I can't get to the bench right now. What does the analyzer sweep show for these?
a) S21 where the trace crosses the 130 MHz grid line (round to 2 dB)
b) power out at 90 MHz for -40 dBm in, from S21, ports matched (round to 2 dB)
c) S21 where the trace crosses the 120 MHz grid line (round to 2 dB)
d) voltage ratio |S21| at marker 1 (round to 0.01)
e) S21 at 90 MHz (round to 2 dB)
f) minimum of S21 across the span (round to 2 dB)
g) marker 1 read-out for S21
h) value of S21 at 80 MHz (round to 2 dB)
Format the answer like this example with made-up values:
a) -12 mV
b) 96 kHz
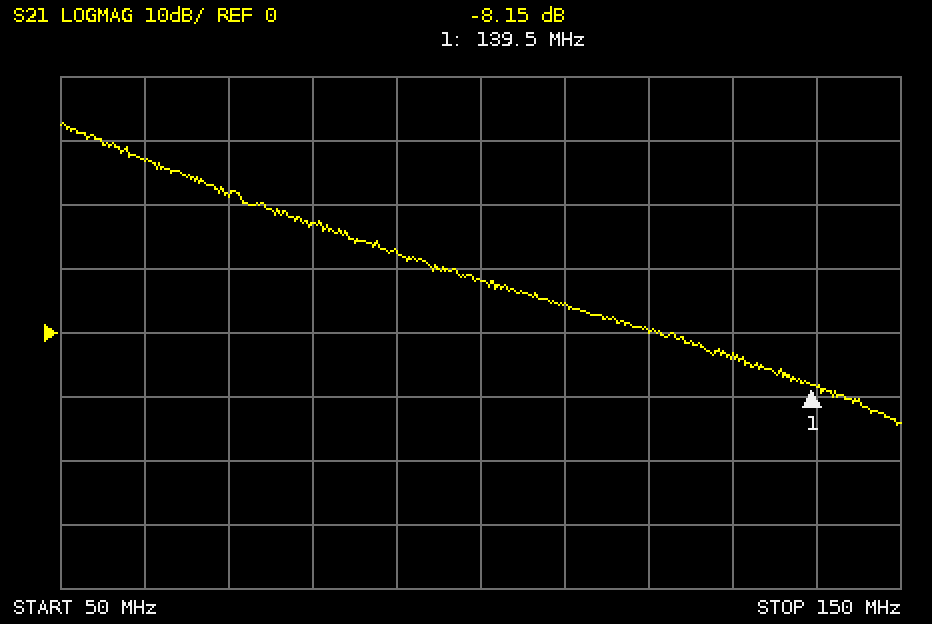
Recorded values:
a) -4 dB
b) -28 dBm
c) 0 dB
d) 0.39
e) 12 dB
f) -14 dB
g) -8.15 dB
h) 18 dB
